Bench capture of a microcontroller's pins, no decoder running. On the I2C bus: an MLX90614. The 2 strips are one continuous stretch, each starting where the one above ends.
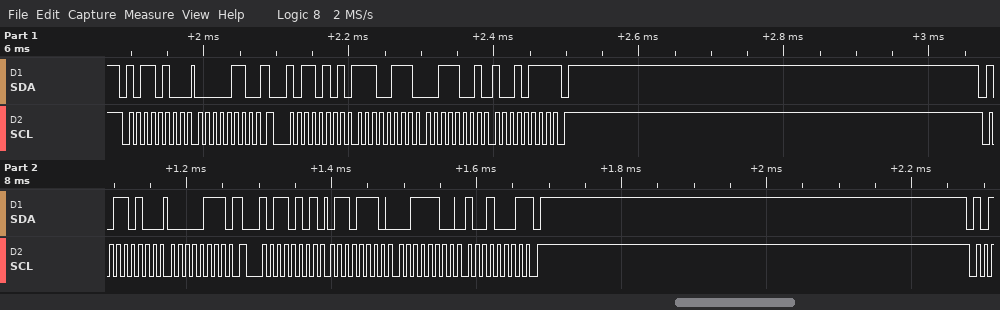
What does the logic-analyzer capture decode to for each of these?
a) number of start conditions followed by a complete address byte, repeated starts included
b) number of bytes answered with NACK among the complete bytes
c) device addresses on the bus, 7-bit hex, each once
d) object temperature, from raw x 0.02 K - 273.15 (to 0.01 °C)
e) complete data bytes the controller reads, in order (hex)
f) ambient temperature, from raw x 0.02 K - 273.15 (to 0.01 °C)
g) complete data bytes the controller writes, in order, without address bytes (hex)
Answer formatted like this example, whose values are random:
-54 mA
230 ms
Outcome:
4
2
0x5A
36.25 °C
E7 39 97 6E 3C 91
23.31 °C
06 07
